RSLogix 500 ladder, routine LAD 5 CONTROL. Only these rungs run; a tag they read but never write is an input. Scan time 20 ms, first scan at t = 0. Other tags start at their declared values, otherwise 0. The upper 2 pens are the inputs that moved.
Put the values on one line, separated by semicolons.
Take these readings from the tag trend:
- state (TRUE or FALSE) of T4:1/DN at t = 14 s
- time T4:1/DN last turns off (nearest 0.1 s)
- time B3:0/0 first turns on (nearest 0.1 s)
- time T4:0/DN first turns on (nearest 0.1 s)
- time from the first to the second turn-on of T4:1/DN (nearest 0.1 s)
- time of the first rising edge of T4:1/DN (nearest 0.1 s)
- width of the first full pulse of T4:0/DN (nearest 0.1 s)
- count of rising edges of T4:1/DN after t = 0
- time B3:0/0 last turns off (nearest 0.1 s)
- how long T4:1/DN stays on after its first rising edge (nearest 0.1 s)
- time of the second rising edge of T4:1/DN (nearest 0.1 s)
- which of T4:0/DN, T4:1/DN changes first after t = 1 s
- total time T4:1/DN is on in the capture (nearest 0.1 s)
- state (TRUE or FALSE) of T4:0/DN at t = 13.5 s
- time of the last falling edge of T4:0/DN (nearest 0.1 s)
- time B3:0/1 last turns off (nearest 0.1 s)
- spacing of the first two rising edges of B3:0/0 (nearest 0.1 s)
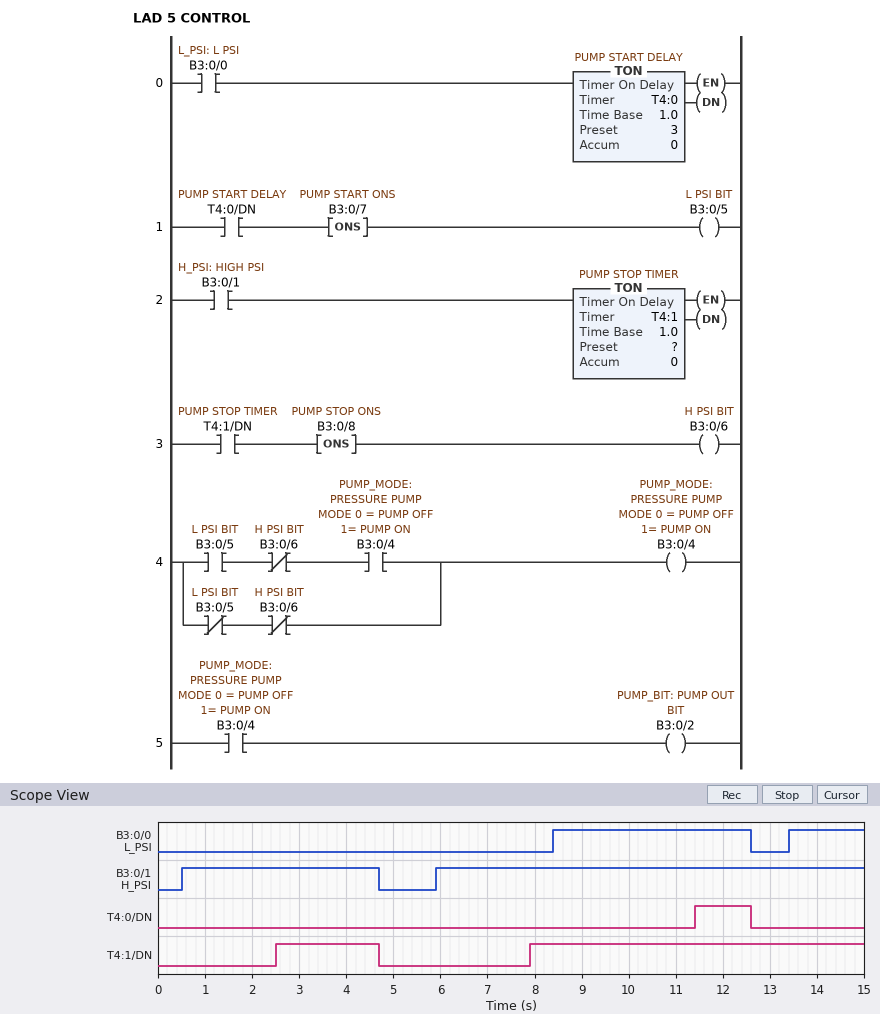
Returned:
TRUE; 4.7 s; 8.4 s; 11.4 s; 5.4 s; 2.5 s; 1.2 s; 2; 12.6 s; 2.2 s; 7.9 s; T4:1/DN; 9.3 s; FALSE; 12.6 s; 4.7 s; 5.0 s
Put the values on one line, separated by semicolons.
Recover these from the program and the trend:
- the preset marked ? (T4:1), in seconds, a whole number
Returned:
2 s
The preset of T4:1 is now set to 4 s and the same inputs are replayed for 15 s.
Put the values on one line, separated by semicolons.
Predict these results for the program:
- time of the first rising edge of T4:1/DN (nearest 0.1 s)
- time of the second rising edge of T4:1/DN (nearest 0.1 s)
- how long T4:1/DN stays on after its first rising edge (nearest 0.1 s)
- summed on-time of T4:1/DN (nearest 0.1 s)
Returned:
4.5 s; 9.9 s; 0.2 s; 5.3 s
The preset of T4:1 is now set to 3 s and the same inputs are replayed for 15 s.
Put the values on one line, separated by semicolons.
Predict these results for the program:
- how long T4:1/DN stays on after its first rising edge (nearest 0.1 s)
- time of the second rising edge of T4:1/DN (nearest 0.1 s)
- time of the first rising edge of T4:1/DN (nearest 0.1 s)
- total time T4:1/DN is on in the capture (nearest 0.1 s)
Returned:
1.2 s; 8.9 s; 3.5 s; 7.3 s
